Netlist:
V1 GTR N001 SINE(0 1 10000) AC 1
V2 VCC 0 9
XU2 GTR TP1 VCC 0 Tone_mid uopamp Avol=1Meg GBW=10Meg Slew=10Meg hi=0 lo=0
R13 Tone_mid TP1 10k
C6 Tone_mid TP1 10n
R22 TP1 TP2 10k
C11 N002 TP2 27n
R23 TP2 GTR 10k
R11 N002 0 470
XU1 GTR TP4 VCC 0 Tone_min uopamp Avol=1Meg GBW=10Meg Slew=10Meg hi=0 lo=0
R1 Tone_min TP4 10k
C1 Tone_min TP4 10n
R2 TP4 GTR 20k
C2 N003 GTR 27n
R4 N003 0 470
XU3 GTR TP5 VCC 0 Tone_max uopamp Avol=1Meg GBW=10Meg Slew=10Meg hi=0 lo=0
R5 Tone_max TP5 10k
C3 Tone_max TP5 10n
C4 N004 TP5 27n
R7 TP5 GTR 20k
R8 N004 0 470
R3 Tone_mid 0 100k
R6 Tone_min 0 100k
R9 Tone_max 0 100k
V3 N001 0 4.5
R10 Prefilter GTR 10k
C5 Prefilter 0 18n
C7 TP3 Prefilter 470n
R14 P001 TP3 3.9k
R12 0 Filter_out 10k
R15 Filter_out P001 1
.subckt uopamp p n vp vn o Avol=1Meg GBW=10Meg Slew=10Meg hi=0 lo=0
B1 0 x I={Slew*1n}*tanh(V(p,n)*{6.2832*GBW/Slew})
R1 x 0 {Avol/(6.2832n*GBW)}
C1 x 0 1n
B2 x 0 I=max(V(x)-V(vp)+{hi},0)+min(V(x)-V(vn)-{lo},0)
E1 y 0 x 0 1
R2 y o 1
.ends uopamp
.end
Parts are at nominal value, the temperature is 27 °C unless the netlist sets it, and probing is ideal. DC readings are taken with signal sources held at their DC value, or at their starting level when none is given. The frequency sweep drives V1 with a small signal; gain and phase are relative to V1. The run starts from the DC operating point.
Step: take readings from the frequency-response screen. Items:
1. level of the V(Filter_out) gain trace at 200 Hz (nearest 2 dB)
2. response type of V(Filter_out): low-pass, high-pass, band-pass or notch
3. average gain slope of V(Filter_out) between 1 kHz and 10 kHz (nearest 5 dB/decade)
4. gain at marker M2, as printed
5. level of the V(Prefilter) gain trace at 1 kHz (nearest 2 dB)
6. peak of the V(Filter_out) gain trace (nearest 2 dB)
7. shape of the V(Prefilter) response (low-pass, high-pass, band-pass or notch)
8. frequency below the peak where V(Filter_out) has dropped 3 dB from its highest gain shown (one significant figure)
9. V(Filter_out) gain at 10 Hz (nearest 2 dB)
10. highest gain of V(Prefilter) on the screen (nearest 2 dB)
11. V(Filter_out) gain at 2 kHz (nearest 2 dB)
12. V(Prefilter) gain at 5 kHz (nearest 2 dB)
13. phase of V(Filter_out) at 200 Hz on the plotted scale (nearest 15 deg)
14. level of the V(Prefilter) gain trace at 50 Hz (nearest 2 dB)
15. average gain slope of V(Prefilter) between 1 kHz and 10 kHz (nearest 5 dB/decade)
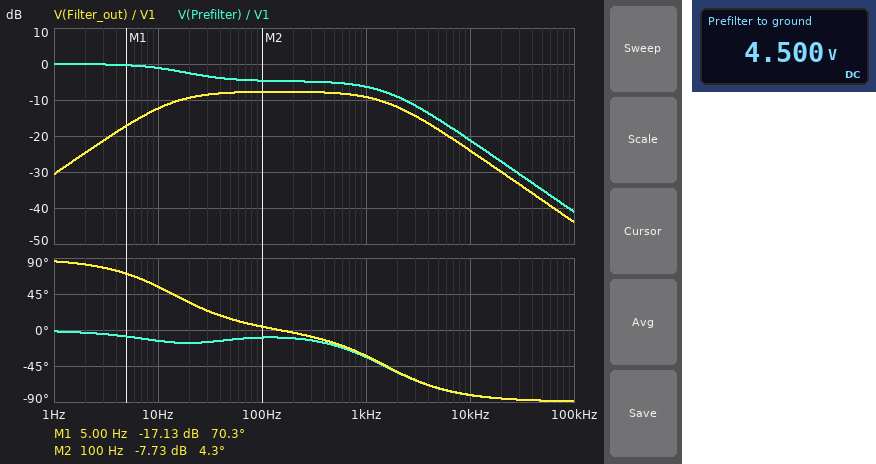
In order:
-8 dB
band-pass
-15 dB/decade
-7.73 dB
-6 dB
-8 dB
low-pass
10 Hz
-12 dB
0 dB
-12 dB
-16 dB
0 deg
-4 dB
-15 dB/decade
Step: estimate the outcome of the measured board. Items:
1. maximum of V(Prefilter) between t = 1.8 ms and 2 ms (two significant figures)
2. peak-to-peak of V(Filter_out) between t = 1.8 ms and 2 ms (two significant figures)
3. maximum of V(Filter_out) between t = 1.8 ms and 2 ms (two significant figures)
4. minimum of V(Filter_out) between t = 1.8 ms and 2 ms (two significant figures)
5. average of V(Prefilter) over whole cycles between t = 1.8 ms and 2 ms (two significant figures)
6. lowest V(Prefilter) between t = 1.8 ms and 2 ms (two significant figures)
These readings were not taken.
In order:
4.6 V
130 mV
62 mV
-63 mV
4.5 V
4.4 V
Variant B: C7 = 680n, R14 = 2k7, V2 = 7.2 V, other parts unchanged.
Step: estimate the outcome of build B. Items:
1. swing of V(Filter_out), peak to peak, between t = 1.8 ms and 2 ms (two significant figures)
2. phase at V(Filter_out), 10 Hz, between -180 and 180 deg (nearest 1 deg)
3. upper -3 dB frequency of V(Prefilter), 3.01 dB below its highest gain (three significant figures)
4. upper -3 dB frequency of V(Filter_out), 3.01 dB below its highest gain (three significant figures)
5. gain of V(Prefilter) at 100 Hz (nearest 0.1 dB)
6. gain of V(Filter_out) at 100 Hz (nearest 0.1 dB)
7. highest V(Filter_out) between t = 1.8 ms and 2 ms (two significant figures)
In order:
140 mV
45 deg
16.6 Hz
1.61 kHz
-5.0 dB
-7.2 dB
68 mV
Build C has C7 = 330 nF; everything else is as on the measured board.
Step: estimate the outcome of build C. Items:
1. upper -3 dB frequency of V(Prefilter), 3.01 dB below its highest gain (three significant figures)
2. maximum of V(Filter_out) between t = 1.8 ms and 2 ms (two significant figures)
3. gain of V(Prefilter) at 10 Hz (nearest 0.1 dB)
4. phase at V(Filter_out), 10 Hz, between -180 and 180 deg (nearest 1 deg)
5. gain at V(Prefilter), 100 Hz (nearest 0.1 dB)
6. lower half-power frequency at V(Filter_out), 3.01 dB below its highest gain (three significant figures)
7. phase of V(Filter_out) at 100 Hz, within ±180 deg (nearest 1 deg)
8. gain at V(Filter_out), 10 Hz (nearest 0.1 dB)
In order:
34.4 Hz
62 mV
-0.6 dB
63 deg
-4.5 dB
19.5 Hz
8 deg
-14.6 dB
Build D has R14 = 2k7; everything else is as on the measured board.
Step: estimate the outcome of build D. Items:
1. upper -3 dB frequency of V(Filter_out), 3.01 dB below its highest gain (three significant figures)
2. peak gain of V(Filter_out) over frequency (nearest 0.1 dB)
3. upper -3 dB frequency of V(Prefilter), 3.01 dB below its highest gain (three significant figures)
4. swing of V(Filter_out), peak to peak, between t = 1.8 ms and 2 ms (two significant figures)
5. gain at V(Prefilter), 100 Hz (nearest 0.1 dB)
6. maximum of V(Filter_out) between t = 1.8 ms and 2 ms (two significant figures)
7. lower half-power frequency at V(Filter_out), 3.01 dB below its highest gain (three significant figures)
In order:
1.62 kHz
-7.3 dB
23.9 Hz
140 mV
-4.9 dB
68 mV
14.5 Hz
